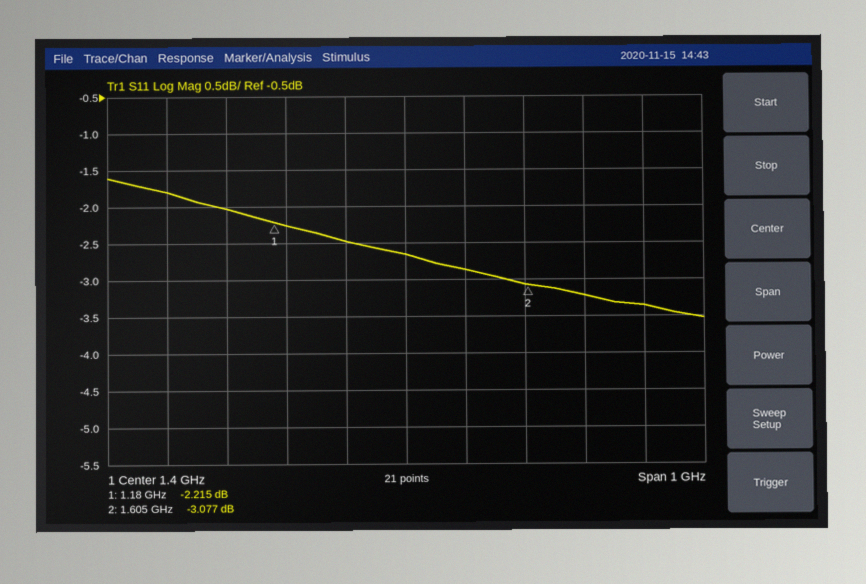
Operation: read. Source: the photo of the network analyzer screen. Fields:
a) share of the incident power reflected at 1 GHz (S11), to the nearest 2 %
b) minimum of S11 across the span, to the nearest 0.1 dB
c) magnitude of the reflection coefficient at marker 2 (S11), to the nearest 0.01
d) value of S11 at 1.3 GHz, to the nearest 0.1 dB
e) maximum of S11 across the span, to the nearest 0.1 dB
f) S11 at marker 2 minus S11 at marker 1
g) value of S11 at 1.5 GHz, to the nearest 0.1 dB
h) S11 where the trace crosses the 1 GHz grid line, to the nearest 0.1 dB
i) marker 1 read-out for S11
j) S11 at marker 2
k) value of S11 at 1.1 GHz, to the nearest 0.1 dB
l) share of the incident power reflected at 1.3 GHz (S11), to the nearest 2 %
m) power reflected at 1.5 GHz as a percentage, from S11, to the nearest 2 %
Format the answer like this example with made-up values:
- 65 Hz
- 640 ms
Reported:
- 66 %
- -3.5 dB
- 0.70
- -2.5 dB
- -1.6 dB
- -0.862 dB
- -2.9 dB
- -1.8 dB
- -2.215 dB
- -3.077 dB
- -2.0 dB
- 56 %
- 52 %
